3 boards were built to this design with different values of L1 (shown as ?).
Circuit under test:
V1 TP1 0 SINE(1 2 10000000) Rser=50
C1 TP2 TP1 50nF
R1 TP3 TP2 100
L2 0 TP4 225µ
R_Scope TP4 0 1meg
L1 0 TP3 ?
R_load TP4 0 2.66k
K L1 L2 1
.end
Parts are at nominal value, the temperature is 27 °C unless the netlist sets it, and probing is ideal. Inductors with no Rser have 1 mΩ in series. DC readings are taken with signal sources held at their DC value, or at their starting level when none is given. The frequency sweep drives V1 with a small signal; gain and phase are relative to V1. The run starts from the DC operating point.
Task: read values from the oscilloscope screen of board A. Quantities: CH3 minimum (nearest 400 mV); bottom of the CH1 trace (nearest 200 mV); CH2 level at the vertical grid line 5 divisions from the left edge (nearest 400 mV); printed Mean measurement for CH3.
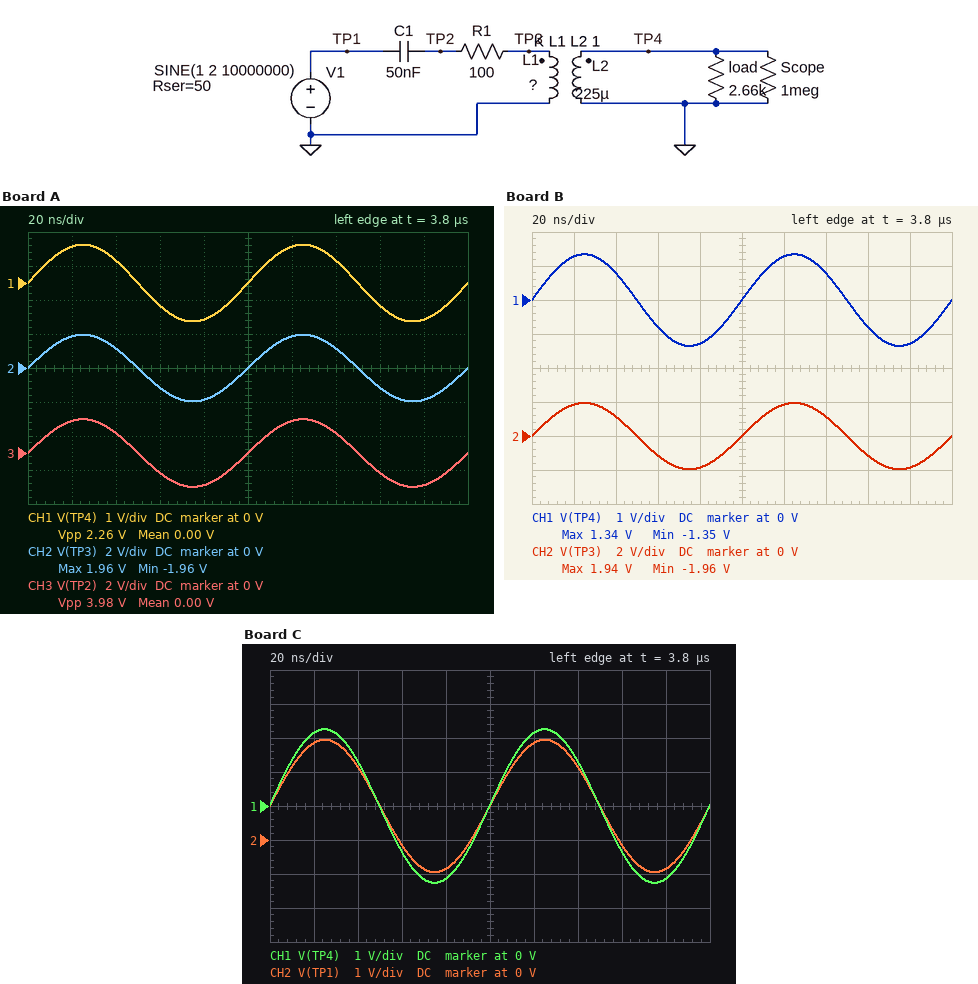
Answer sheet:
-2.0 V
-1.2 V
0 V
0.00 V
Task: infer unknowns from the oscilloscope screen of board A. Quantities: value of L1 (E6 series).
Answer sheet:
680 µH
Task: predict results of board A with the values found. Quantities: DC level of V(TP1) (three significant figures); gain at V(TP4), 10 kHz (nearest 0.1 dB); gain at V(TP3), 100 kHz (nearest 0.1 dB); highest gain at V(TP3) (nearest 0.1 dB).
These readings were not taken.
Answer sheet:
1.00 V
-22.1 dB
-0.1 dB
0 dB
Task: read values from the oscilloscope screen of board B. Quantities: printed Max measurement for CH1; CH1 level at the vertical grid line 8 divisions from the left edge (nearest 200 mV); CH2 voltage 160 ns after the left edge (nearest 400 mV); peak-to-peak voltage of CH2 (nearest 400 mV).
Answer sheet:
1.34 V
-800 mV
-1.2 V
4.0 V
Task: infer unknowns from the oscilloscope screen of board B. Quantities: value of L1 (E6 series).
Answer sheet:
470 µH
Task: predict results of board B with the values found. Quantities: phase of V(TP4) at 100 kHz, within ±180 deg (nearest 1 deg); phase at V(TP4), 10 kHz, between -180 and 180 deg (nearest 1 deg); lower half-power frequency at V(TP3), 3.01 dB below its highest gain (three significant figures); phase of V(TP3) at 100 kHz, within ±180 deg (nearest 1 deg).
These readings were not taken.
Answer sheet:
29 deg
152 deg
35.6 kHz
29 deg
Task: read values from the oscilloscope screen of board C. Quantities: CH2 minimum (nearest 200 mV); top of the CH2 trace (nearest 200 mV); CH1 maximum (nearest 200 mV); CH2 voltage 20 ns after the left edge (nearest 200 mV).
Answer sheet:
-1.0 V
3.0 V
2.2 V
2.8 V
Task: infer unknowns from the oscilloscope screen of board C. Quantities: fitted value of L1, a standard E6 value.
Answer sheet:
150 µH
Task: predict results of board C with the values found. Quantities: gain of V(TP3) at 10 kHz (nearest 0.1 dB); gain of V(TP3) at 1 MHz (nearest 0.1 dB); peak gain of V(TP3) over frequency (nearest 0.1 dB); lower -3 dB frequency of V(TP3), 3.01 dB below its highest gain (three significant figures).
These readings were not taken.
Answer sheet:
-31.2 dB
-0.8 dB
-0.7 dB
128 kHz
